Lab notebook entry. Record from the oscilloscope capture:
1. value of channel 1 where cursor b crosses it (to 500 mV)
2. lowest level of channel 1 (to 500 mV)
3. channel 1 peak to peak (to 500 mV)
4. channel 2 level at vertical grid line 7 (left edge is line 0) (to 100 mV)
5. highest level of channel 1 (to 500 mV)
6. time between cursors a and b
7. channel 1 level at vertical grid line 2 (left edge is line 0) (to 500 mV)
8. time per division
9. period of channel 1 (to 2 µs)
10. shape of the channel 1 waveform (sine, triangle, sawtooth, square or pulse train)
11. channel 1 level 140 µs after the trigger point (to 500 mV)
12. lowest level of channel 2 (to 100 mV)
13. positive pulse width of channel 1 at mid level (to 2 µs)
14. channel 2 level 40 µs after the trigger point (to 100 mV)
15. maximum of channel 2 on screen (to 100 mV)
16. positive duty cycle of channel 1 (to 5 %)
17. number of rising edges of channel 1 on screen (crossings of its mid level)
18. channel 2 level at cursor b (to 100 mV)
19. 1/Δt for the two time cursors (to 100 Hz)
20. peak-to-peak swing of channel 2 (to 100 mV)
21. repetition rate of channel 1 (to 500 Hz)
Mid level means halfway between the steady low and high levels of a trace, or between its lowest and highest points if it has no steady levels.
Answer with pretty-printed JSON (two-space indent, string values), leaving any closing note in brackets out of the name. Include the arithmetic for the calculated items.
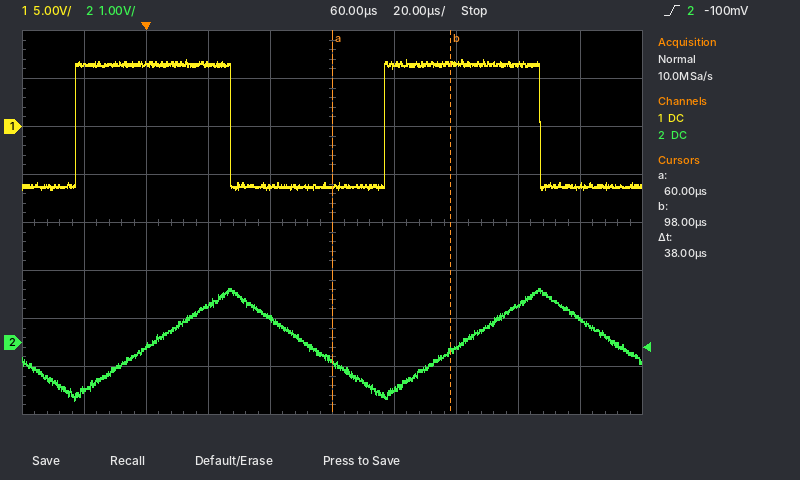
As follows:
{
  "value of channel 1 where cursor b crosses it": "6.5 V",
  "lowest level of channel 1": "-6.5 V",
  "channel 1 peak to peak": "7.0 V − (-6.5 V) = 13.5 V",
  "channel 2 level at vertical grid line 7 (left edge is line 0)": "-100 mV",
  "highest level of channel 1": "7.0 V",
  "time between cursors a and b": "38 µs",
  "channel 1 level at vertical grid line 2 (left edge is line 0)": "6.5 V",
  "time per division": "20 µs",
  "period of channel 1": "100 µs",
  "shape of the channel 1 waveform": "square",
  "channel 1 level 140 µs after the trigger point": "-6.0 V",
  "lowest level of channel 2": "-1.2 V",
  "positive pulse width of channel 1 at mid level": "50 µs",
  "channel 2 level 40 µs after the trigger point": "500 mV",
  "maximum of channel 2 on screen": "1.1 V",
  "positive duty cycle of channel 1": "50 µs / 100 µs ≈ 50 %",
  "number of rising edges of channel 1 on screen": "2",
  "channel 2 level at cursor b": "-200 mV",
  "1/Δt for the two time cursors": "1 / 38 µs ≈ 26.3 kHz",
  "peak-to-peak swing of channel 2": "1.1 V − (-1.2 V) = 2.3 V",
  "repetition rate of channel 1": "1 / 100 µs ≈ 10.0 kHz"
}
